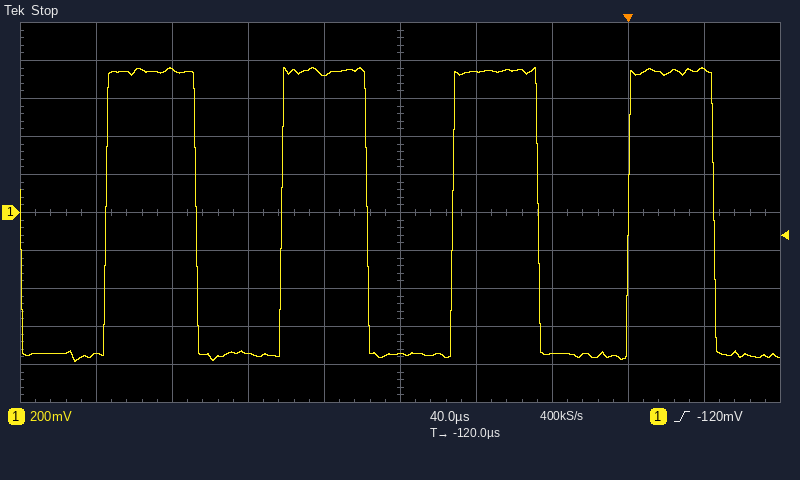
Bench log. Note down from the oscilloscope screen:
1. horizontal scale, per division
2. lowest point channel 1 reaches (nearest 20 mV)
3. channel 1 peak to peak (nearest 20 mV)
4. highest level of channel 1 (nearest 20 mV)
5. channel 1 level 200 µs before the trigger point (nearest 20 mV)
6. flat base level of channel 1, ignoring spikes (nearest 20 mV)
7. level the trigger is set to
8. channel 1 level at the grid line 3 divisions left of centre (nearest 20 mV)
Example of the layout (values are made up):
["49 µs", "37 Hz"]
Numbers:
["40 µs", "-780 mV", "1.54 V", "760 mV", "-740 mV", "-740 mV", "-120 mV", "760 mV"]
